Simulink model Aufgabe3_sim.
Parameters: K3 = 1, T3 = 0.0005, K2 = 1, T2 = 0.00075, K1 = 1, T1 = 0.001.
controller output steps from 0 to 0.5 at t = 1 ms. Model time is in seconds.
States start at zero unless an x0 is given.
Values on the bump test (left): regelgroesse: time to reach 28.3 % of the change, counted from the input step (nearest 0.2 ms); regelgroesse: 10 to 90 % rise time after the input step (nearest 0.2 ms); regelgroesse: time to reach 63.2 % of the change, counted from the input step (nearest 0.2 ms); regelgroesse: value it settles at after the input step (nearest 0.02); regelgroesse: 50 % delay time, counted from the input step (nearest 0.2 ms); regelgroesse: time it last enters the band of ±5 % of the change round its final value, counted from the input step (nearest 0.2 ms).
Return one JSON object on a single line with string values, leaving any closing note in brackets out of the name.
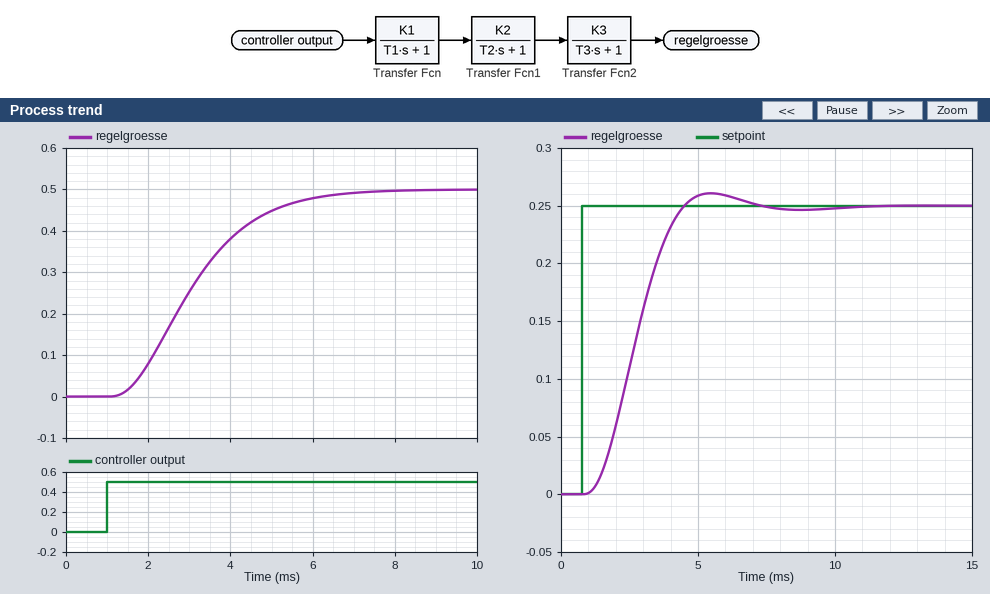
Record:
{"regelgroesse: time to reach 28.3 % of the change, counted from the input step": "1.4 ms", "regelgroesse: 10 to 90 % rise time after the input step": "3.2 ms", "regelgroesse: time to reach 63.2 % of the change, counted from the input step": "2.4 ms", "regelgroesse: value it settles at after the input step": "0.50", "regelgroesse: 50 % delay time, counted from the input step": "2.0 ms", "regelgroesse: time it last enters the band of ±5 % of the change round its final value, counted from the input step": "4.8 ms"}
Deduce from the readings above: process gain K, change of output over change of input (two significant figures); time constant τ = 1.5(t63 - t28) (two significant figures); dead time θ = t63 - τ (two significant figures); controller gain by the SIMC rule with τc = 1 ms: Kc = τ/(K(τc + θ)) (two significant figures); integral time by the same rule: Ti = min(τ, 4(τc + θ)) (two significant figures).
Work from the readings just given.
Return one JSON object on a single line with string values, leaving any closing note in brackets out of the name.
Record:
{"process gain K, change of output over change of input": "1.0", "time constant τ = 1.5(t63 - t28)": "1.5 ms", "dead time θ = t63 - τ": "0.90 ms", "controller gain by the SIMC rule with τc = 1 ms: Kc = τ/(K(τc + θ))": "0.79", "integral time by the same rule: Ti = min(τ, 4(τc + θ))": "1.5 ms"}
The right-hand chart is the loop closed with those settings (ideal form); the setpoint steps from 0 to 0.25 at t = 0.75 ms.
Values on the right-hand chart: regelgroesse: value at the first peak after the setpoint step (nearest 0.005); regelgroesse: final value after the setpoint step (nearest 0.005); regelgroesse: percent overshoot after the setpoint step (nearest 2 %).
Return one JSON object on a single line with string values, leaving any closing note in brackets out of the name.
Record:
{"regelgroesse: value at the first peak after the setpoint step": "0.260", "regelgroesse: final value after the setpoint step": "0.250", "regelgroesse: percent overshoot after the setpoint step": "4 %"}
